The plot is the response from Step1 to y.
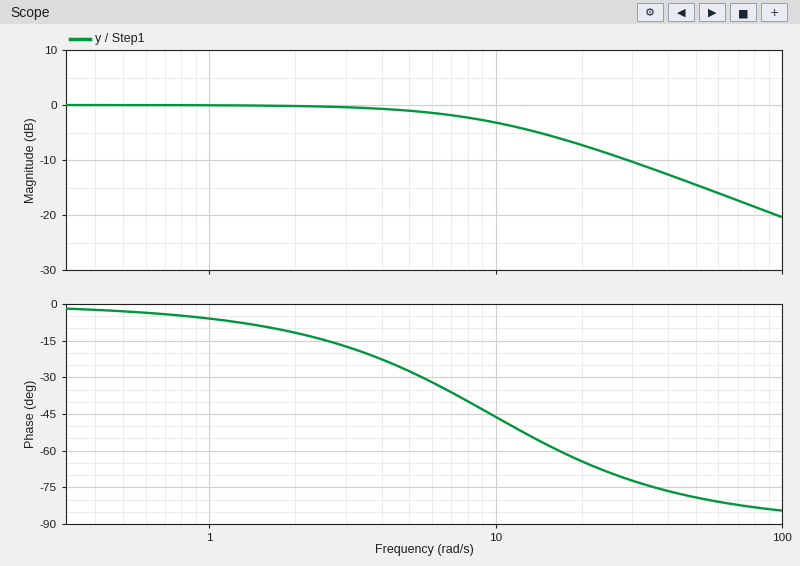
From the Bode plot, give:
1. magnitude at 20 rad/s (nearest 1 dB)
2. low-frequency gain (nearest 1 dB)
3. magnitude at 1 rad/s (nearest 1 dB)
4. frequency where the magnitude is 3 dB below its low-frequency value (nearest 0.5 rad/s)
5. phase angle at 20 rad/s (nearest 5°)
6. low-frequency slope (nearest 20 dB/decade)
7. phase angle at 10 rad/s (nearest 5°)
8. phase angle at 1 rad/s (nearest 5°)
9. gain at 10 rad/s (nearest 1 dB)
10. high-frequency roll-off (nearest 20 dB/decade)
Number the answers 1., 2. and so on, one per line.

1. -7 dB
2. 0 dB
3. 0 dB
4. 9.5 rad/s
5. -65°
6. 0 dB/decade
7. -45°
8. -5°
9. -3 dB
10. -20 dB/decade
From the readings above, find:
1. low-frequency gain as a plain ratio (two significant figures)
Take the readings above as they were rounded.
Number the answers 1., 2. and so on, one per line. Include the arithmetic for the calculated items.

1. 10^(0 / 20) = 1.0
